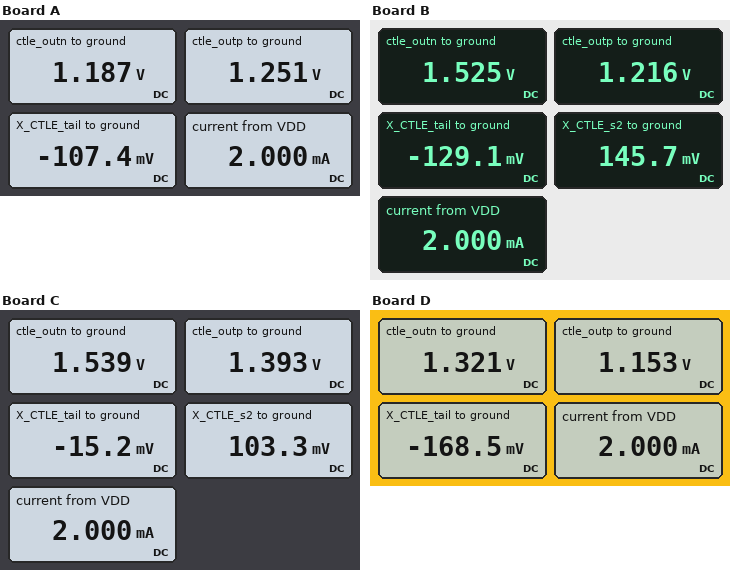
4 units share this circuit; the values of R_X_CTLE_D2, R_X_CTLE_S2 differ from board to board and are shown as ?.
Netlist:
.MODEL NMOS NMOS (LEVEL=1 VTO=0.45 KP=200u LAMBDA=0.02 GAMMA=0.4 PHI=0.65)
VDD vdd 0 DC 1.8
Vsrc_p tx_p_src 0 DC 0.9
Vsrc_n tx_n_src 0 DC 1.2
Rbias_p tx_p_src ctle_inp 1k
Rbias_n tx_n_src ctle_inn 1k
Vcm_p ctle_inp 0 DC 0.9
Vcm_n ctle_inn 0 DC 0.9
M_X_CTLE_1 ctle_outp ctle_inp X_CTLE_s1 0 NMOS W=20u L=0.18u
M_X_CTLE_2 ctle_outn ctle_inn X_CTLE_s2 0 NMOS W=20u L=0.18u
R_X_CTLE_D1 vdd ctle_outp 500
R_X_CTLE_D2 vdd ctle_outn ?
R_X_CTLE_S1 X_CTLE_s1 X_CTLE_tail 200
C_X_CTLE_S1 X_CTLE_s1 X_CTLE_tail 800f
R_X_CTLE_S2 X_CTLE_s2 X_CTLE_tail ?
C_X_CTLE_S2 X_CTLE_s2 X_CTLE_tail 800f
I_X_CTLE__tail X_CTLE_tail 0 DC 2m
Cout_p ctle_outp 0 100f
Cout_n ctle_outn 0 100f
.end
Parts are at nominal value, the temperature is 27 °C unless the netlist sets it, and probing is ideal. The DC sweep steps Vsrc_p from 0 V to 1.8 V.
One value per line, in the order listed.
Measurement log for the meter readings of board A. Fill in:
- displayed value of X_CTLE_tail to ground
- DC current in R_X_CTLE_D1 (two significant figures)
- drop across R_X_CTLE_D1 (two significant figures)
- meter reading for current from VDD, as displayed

-107.4 mV
1.1 mA
550 mV
2.000 mA
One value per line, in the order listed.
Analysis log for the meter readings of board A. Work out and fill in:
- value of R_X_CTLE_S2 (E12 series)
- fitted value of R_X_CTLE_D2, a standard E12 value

270 Ω
680 Ω
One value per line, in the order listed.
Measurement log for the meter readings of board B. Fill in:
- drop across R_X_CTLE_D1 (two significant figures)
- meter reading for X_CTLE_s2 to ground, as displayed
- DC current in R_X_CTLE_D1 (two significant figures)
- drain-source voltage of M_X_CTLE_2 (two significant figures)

580 mV
145.7 mV
1.2 mA
1.4 V
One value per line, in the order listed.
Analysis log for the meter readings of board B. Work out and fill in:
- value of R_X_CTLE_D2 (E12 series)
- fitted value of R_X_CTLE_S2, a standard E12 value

330 Ω
330 Ω
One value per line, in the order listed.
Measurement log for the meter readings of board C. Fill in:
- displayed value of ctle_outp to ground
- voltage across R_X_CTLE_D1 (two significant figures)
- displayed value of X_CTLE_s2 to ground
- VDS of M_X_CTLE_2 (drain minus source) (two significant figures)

1.393 V
410 mV
103.3 mV
1.4 V
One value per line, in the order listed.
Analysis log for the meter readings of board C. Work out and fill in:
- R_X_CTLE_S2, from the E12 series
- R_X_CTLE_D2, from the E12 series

100 Ω
220 Ω
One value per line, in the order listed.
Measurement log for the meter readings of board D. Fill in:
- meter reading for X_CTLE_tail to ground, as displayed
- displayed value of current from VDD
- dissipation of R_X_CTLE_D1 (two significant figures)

-168.5 mV
2.000 mA
840 µW
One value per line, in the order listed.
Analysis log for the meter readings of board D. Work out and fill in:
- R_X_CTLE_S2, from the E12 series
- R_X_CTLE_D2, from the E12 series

470 Ω
680 Ω
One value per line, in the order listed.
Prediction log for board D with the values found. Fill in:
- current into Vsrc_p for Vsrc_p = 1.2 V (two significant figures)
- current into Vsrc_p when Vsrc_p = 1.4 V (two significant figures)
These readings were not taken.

-300 µA
-500 µA
